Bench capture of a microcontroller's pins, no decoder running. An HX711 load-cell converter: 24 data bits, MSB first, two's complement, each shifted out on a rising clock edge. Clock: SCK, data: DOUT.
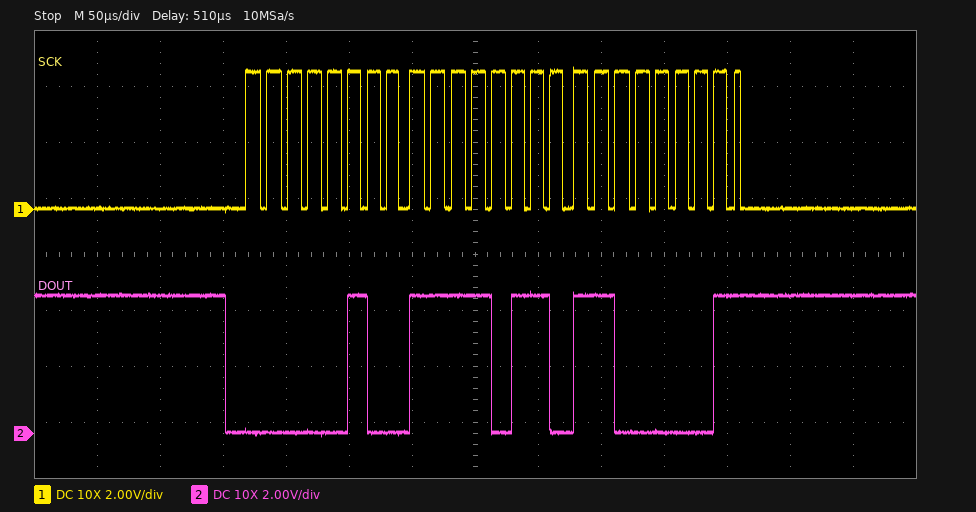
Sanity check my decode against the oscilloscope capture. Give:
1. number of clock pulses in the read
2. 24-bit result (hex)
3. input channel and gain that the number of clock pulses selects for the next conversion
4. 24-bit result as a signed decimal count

25
0x04F6C1
channel A, gain 128
325313
